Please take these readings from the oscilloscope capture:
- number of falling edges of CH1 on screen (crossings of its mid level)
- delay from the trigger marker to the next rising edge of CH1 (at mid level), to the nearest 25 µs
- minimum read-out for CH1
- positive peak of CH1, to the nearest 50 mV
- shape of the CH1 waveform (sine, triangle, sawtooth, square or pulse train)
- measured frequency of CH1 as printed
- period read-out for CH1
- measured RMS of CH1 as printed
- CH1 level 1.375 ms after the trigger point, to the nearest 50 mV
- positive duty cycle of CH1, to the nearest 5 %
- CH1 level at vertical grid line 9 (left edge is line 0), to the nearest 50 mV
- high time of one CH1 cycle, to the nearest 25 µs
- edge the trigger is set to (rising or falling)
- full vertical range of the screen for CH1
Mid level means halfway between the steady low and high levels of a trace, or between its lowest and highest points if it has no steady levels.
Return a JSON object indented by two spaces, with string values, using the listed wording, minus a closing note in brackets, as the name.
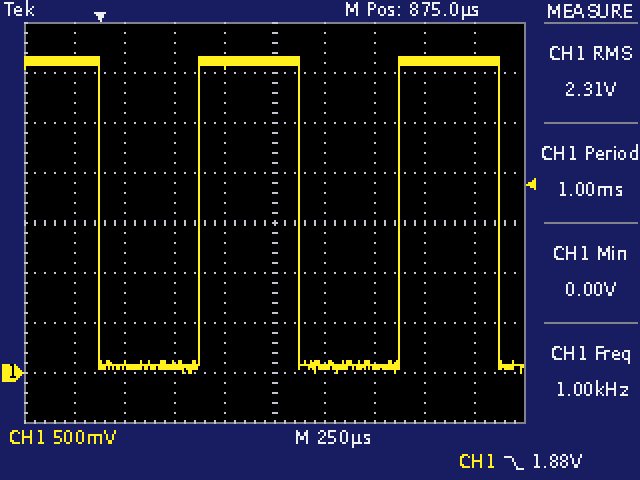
{
  "number of falling edges of CH1 on screen": "3",
  "delay from the trigger marker to the next rising edge of CH1 (at mid level), to the nearest 25 µs": "500 µs",
  "minimum read-out for CH1": "0.00 V",
  "positive peak of CH1, to the nearest 50 mV": "3.15 V",
  "shape of the CH1 waveform": "square",
  "measured frequency of CH1 as printed": "1.00 kHz",
  "period read-out for CH1": "1.00 ms",
  "measured RMS of CH1 as printed": "2.31 V",
  "CH1 level 1.375 ms after the trigger point, to the nearest 50 mV": "50 mV",
  "positive duty cycle of CH1, to the nearest 5 %": "50 %",
  "CH1 level at vertical grid line 9 (left edge is line 0), to the nearest 50 mV": "3.10 V",
  "high time of one CH1 cycle, to the nearest 25 µs": "500 µs",
  "edge the trigger is set to": "falling",
  "full vertical range of the screen for CH1": "4 V"
}
